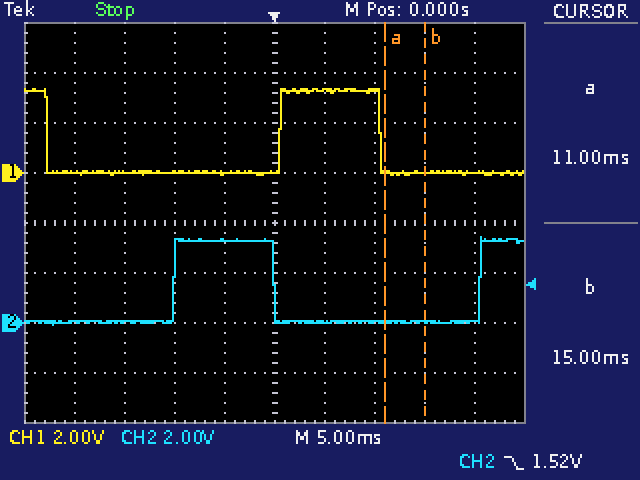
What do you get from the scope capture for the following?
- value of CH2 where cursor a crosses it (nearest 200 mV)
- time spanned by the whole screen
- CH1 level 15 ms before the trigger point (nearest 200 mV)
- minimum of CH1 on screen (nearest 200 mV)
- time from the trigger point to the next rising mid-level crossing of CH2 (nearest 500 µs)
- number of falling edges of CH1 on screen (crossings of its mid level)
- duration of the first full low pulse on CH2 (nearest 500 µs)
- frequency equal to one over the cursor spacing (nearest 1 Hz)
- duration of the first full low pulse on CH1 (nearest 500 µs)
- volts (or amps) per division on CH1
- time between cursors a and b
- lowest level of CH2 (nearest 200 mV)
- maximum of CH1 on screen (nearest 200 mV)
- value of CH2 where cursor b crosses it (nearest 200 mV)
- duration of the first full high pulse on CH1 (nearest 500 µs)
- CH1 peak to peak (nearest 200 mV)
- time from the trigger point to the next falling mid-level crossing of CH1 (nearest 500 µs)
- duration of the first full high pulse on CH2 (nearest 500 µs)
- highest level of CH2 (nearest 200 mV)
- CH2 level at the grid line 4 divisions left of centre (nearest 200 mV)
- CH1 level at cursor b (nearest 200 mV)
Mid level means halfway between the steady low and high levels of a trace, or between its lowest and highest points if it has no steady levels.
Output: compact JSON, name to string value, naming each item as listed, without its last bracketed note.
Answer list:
{"value of CH2 where cursor a crosses it": "0.0 V", "time spanned by the whole screen": "50 ms", "CH1 level 15 ms before the trigger point": "0.0 V", "minimum of CH1 on screen": "0.0 V", "time from the trigger point to the next rising mid-level crossing of CH2": "20.5 ms", "number of falling edges of CH1 on screen": "2", "duration of the first full low pulse on CH2": "20.5 ms", "frequency equal to one over the cursor spacing": "250 Hz", "duration of the first full low pulse on CH1": "23.5 ms", "volts (or amps) per division on CH1": "2 V", "time between cursors a and b": "4.0 ms", "lowest level of CH2": "0.0 V", "maximum of CH1 on screen": "3.4 V", "value of CH2 where cursor b crosses it": "0.0 V", "duration of the first full high pulse on CH1": "10.0 ms", "CH1 peak to peak": "3.4 V", "time from the trigger point to the next falling mid-level crossing of CH1": "10.5 ms", "duration of the first full high pulse on CH2": "10.0 ms", "highest level of CH2": "3.4 V", "CH2 level at the grid line 4 divisions left of centre": "0.0 V", "CH1 level at cursor b": "0.0 V"}
